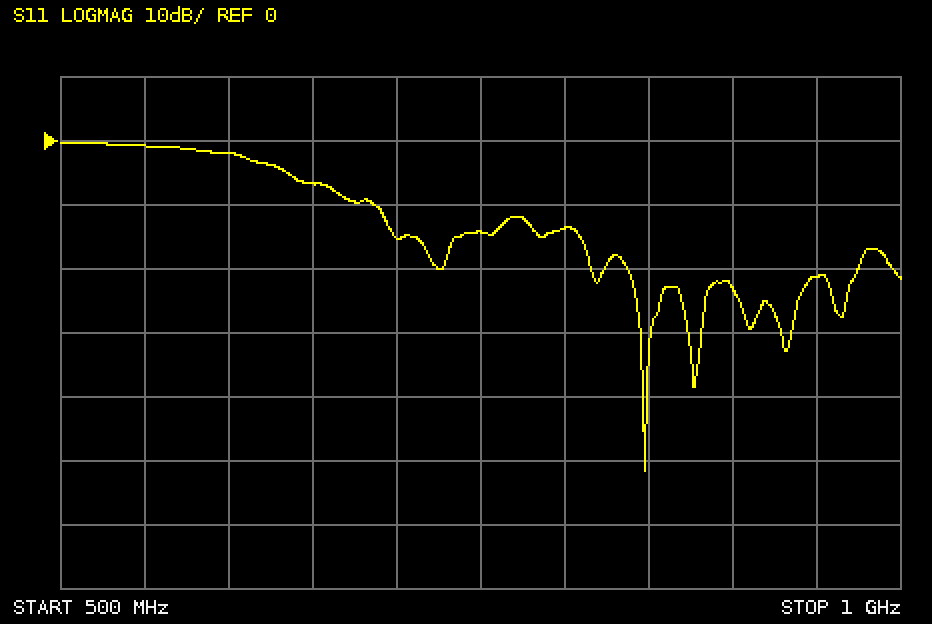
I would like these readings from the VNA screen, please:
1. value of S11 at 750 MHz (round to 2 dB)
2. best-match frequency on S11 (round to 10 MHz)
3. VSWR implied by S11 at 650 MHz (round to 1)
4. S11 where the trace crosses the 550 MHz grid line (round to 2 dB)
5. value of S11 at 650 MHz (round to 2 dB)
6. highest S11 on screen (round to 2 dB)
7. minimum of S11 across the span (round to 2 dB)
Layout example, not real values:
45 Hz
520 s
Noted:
-14 dB
850 MHz
3
0 dB
-6 dB
0 dB
-52 dB
